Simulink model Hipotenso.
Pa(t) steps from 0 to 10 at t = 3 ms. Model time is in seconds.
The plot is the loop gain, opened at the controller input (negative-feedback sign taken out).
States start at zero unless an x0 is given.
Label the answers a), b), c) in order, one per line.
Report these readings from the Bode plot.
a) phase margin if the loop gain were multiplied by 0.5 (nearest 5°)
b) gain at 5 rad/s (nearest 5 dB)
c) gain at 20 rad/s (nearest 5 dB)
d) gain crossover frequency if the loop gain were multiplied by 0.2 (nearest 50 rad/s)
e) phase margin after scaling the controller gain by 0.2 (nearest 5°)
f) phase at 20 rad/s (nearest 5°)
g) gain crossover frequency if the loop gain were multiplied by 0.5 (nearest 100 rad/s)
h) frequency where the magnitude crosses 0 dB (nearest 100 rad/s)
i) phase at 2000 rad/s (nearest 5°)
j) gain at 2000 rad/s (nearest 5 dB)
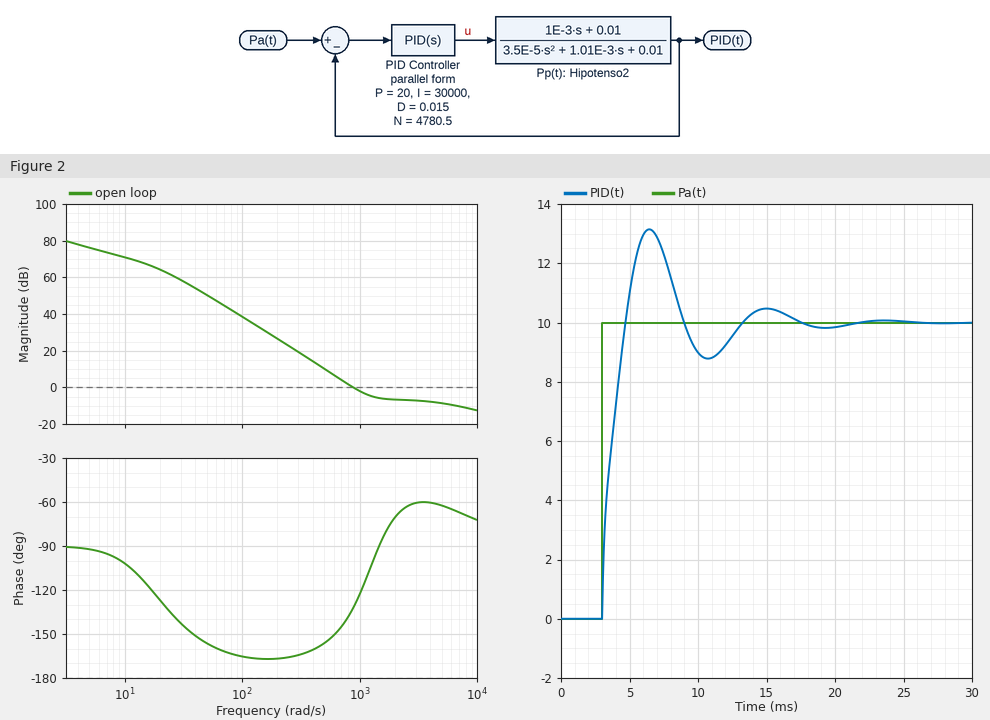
a) 30°
b) 75 dB
c) 65 dB
d) 400 rad/s
e) 20°
f) -125°
g) 600 rad/s
h) 900 rad/s
i) -70°
j) -5 dB
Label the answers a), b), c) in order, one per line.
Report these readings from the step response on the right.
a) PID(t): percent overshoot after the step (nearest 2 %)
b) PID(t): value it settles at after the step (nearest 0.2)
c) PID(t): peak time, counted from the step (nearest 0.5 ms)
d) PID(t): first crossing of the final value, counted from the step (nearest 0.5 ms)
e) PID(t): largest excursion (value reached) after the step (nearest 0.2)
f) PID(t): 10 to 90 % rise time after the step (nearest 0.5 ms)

a) 32 %
b) 10.0
c) 3.5 ms
d) 1.5 ms
e) 13.2
f) 1.5 ms
